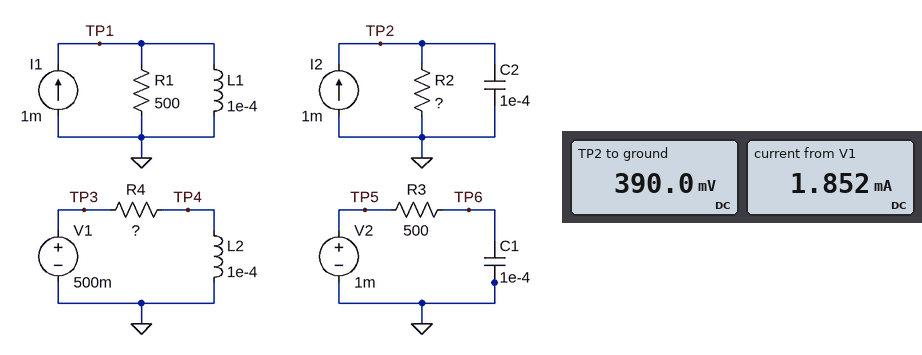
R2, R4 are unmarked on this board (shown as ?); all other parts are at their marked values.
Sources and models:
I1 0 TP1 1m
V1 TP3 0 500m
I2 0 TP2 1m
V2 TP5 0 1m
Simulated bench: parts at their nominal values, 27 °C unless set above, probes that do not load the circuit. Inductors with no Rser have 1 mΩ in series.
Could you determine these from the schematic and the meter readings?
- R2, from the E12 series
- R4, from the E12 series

390 Ω
270 Ω
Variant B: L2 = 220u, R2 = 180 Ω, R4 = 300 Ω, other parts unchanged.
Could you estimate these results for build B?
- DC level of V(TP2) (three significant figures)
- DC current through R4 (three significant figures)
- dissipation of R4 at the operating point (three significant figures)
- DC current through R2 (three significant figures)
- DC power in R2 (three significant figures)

180 mV
1.67 mA
833 µW
1.00 mA
180 µW
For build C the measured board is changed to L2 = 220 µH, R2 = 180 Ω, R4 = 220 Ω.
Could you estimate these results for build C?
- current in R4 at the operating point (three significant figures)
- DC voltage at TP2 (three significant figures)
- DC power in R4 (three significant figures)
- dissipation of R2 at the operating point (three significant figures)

2.27 mA
180 mV
1.14 mW
180 µW
